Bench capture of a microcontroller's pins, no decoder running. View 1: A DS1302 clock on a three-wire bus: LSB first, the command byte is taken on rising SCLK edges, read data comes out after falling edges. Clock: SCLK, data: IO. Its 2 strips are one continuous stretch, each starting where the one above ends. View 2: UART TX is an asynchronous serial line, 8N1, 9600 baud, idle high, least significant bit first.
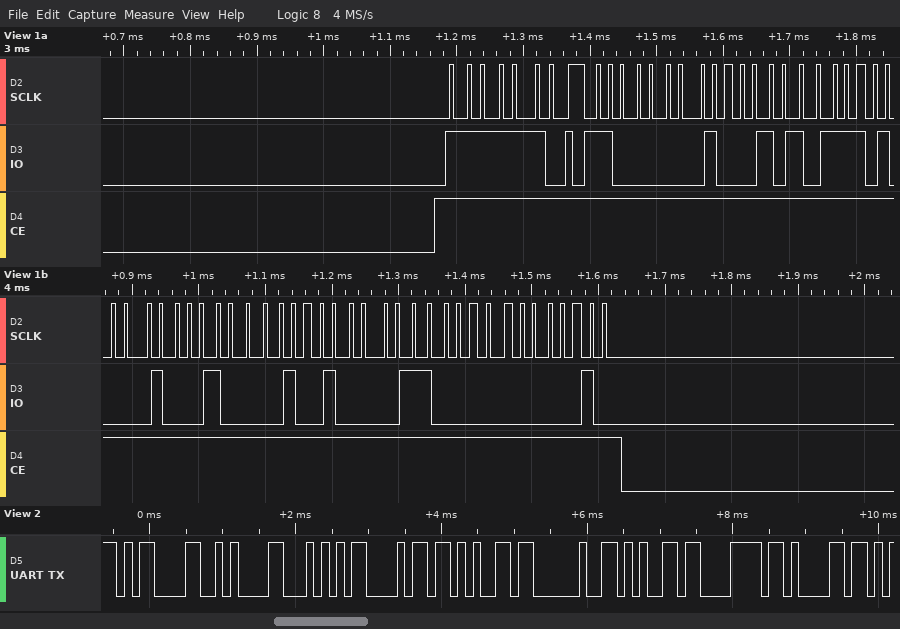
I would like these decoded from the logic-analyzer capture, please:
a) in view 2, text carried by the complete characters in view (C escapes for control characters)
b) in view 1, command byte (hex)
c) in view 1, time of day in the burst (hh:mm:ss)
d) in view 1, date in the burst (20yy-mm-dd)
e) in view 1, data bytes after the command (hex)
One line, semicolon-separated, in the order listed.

"\r\nThe exa"; 0xBF; 17:51:03; 2020-12-11; 03 51 17 11 12 06 20
